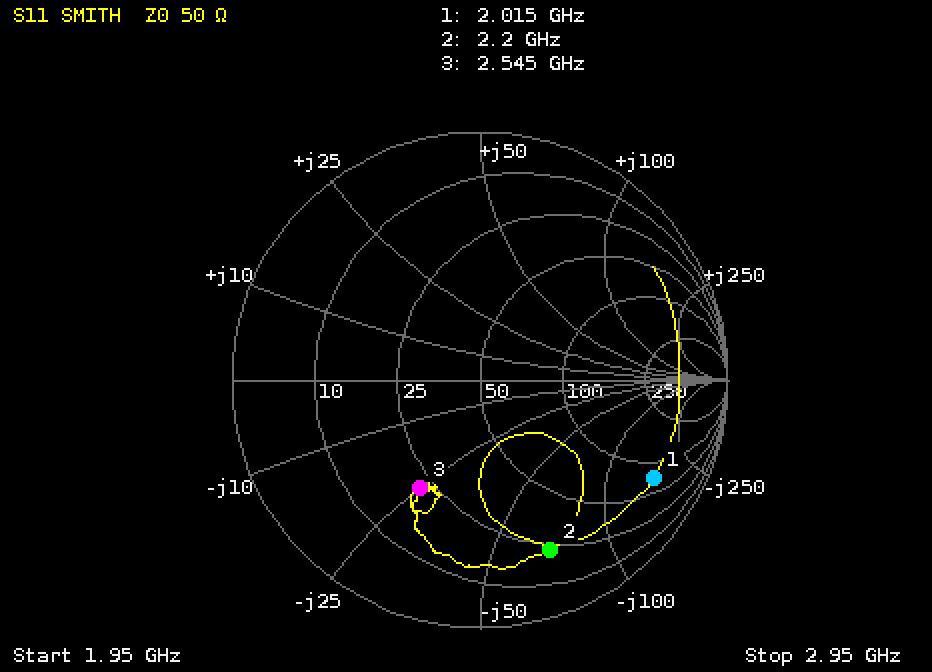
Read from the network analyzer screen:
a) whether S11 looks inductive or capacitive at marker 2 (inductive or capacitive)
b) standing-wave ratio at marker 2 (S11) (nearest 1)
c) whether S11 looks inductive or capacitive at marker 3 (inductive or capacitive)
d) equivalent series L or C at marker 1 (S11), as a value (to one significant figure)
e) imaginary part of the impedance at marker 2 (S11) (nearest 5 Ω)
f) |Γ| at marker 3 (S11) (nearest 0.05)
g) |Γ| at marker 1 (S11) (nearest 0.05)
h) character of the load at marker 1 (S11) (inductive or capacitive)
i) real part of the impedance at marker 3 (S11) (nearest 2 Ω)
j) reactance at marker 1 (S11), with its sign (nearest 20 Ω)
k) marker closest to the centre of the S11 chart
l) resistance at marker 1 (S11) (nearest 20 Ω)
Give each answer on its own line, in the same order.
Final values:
capacitive
7
capacitive
500 fF
-70 Ω
0.50
0.80
capacitive
22 Ω
-160 Ω
marker 3
80 Ω
